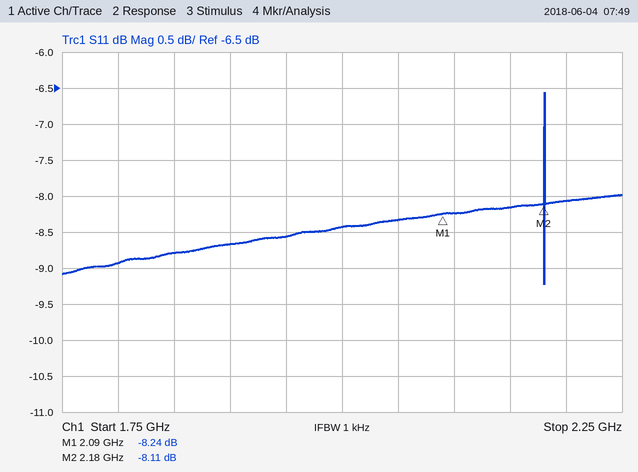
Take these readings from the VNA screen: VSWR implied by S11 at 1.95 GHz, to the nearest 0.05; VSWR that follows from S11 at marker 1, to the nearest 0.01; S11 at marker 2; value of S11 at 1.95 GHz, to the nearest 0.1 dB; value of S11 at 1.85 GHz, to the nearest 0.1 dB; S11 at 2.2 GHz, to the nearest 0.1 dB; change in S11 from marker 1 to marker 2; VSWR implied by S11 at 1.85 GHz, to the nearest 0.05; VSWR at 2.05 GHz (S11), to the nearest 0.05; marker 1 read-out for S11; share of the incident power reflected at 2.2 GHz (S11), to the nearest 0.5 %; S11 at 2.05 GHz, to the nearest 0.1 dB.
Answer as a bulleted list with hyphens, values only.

- 2.20
- 2.26
- -8.11 dB
- -8.6 dB
- -8.8 dB
- -8.1 dB
- 0.13 dB
- 2.15
- 2.25
- -8.24 dB
- 15.5 %
- -8.3 dB
